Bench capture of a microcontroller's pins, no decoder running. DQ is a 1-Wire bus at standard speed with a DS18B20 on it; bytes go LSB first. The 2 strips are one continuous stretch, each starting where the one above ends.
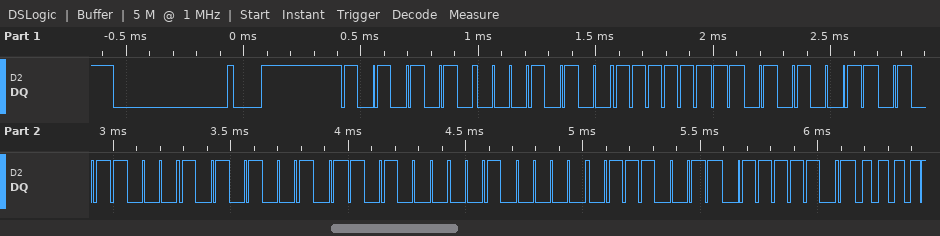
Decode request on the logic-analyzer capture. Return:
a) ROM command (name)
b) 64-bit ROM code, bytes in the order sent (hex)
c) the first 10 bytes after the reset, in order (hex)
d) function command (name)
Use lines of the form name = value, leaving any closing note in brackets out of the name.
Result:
ROM command = Match ROM
64-bit ROM code, bytes in the order sent = 28 FF CA 1A 95 16 04 CE
the first 10 bytes after the reset, in order = 55 28 FF CA 1A 95 16 04 CE BE
function command = Read Scratchpad
